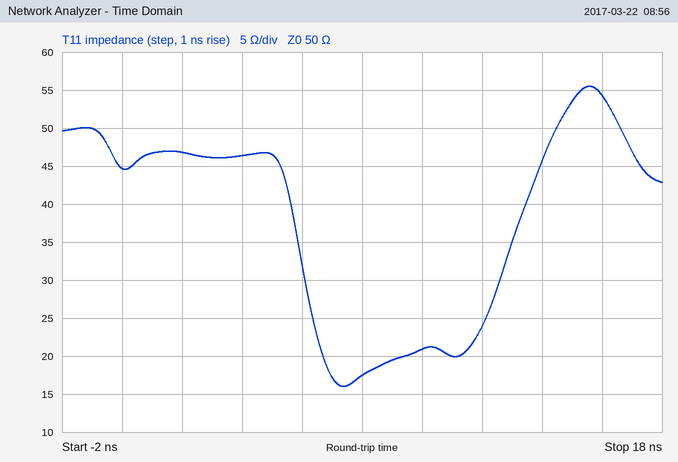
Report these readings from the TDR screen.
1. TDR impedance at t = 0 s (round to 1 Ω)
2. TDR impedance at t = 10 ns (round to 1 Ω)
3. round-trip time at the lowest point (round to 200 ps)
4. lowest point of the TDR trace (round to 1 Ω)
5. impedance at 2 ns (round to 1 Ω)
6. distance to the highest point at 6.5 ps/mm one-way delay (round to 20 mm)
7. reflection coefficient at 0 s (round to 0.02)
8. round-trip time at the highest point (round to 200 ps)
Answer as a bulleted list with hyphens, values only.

- 45 Ω
- 21 Ω
- 7.4 ns
- 16 Ω
- 47 Ω
- 1.20 m
- -0.06
- 15.6 ns
